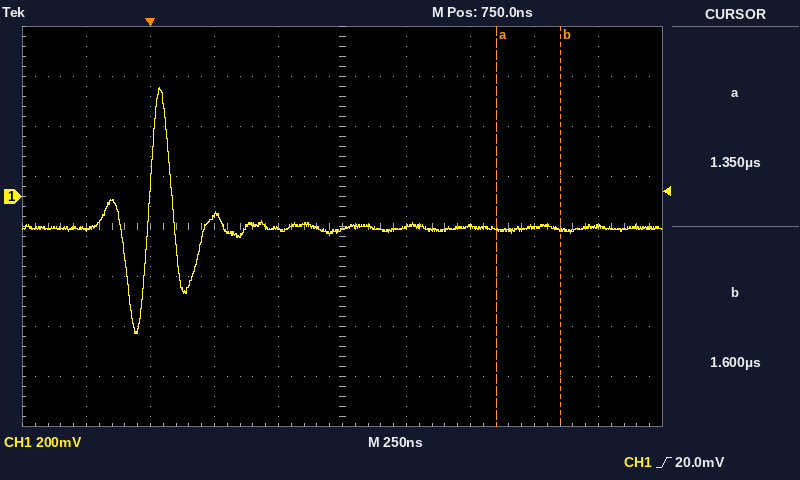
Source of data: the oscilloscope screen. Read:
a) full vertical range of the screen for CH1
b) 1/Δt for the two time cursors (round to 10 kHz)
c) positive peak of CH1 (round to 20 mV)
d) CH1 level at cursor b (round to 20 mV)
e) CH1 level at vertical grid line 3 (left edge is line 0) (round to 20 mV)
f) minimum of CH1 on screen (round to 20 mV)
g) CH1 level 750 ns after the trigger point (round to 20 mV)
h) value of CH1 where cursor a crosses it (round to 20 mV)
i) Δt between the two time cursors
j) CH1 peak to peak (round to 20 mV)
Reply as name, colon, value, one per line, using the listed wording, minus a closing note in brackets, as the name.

full vertical range of the screen for CH1: 1.6 V
1/Δt for the two time cursors: 4.00 MHz
positive peak of CH1: 440 mV
CH1 level at cursor b: -140 mV
CH1 level at vertical grid line 3 (left edge is line 0): -80 mV
minimum of CH1 on screen: -540 mV
CH1 level 750 ns after the trigger point: -140 mV
value of CH1 where cursor a crosses it: -140 mV
Δt between the two time cursors: 250 ns
CH1 peak to peak: 980 mV
